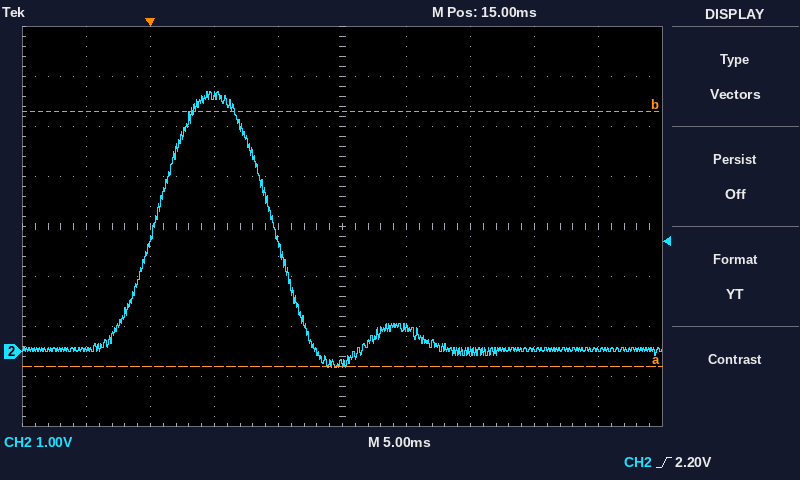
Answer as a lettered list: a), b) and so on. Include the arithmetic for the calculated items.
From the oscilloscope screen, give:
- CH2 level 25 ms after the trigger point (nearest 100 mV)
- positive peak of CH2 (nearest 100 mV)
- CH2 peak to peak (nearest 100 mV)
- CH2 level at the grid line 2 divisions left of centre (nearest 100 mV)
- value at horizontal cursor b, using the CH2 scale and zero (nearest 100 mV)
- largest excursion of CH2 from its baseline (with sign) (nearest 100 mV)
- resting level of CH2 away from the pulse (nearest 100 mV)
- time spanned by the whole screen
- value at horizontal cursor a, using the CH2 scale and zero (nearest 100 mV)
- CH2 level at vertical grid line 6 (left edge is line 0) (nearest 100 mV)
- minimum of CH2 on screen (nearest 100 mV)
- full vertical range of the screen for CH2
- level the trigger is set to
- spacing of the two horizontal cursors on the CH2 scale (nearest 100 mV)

a) 0.0 V
b) 5.2 V
c) 5.2 V − (-300 mV) = 5.5 V
d) 5.1 V
e) 4.8 V
f) 5.2 V − (0.0 V) = +5.2 V
g) 0.0 V
h) 50 ms
i) -300 mV
j) 500 mV
k) -300 mV
l) 8 V
m) 2.20 V
n) 5.1 V
